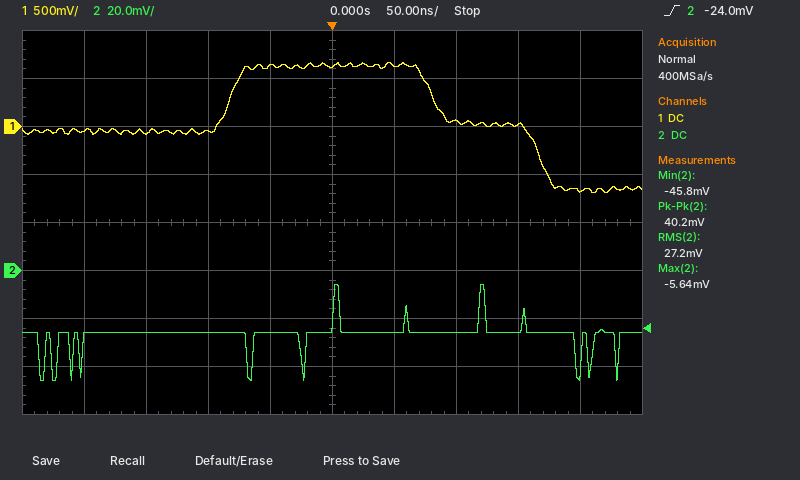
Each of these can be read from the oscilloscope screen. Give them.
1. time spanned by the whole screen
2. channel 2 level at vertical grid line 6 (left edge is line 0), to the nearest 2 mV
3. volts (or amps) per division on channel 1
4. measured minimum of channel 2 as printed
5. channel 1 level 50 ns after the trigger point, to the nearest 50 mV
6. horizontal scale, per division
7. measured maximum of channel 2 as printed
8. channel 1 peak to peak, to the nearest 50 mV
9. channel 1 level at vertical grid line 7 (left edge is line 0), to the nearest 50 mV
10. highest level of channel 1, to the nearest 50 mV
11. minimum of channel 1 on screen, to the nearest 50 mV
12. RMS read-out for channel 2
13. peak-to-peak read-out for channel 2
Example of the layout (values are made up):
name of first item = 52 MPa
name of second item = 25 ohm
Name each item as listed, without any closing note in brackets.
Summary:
time spanned by the whole screen = 500 ns
channel 2 level at vertical grid line 6 (left edge is line 0), to the nearest 2 mV = -26 mV
volts (or amps) per division on channel 1 = 500 mV
measured minimum of channel 2 as printed = -45.8 mV
channel 1 level 50 ns after the trigger point, to the nearest 50 mV = 650 mV
horizontal scale, per division = 50 ns
measured maximum of channel 2 as printed = -5.64 mV
channel 1 peak to peak, to the nearest 50 mV = 1.35 V
channel 1 level at vertical grid line 7 (left edge is line 0), to the nearest 50 mV = 50 mV
highest level of channel 1, to the nearest 50 mV = 650 mV
minimum of channel 1 on screen, to the nearest 50 mV = -700 mV
RMS read-out for channel 2 = 27.2 mV
peak-to-peak read-out for channel 2 = 40.2 mV
